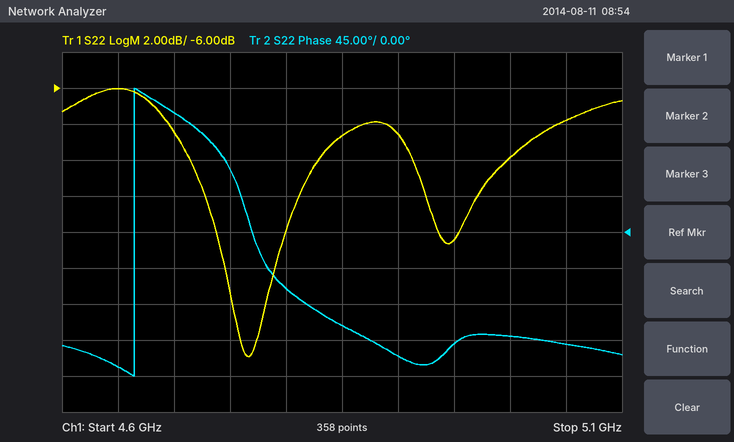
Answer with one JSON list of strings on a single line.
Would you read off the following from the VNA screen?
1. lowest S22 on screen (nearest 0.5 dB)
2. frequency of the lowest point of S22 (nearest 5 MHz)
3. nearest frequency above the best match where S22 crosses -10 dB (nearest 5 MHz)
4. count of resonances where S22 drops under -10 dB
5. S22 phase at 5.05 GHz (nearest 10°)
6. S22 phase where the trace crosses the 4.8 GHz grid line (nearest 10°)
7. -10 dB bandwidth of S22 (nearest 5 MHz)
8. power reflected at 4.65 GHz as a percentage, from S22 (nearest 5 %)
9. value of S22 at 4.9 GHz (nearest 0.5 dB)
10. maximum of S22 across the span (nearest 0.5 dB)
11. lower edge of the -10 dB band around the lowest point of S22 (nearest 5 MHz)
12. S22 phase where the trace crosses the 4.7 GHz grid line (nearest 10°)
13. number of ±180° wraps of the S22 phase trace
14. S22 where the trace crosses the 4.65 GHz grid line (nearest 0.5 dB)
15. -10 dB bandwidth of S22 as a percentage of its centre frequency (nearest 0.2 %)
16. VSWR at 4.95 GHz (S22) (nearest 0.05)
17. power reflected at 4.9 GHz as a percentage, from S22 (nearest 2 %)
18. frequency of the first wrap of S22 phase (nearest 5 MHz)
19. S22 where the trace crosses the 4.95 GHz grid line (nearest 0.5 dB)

["-21.0 dB", "4.765 GHz", "4.830 GHz", "2", "-140°", "-70°", "115 MHz", "25 %", "-8.5 dB", "-6.0 dB", "4.715 GHz", "150°", "1", "-6.0 dB", "2.4 %", "1.45", "14 %", "4.665 GHz", "-14.5 dB"]
